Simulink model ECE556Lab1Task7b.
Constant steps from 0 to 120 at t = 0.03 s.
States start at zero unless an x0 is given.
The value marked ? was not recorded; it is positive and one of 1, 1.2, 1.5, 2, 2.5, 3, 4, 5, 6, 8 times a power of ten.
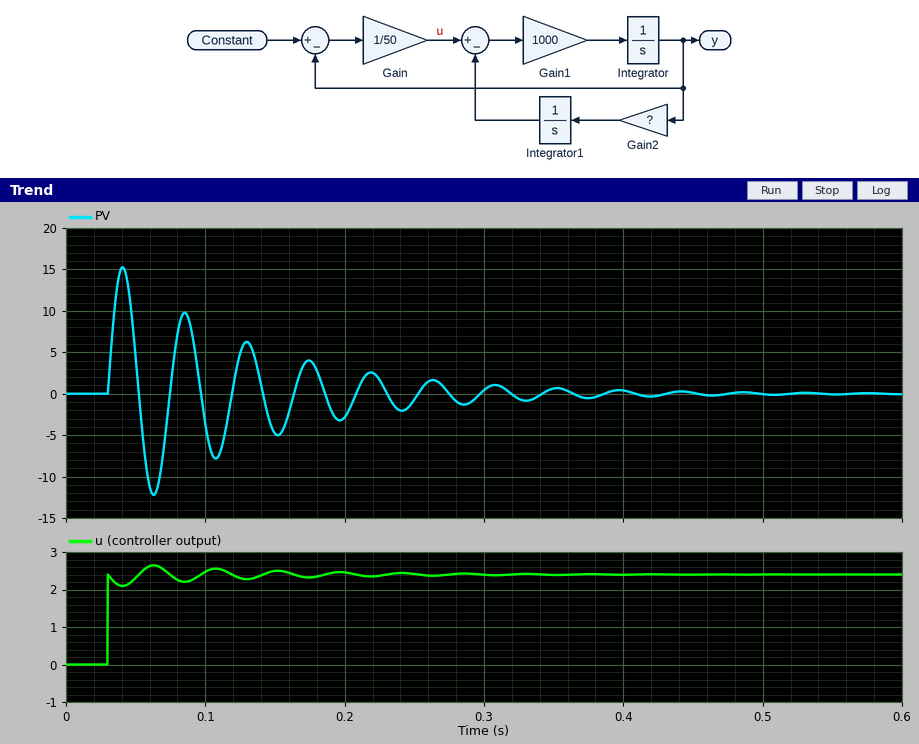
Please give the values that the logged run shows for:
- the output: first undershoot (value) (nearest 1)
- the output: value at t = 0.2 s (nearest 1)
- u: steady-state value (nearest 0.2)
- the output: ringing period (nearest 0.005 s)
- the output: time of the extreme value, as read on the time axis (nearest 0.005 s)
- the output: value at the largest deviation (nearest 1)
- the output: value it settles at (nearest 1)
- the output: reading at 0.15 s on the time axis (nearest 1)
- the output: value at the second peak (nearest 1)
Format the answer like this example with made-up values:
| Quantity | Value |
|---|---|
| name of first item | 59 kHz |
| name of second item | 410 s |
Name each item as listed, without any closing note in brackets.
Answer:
| Quantity | Value |
|---|---|
| the output: first undershoot (value) | -12 |
| the output: value at t = 0.2 s | -3 |
| u: steady-state value | 2.4 |
| the output: ringing period | 0.045 s |
| the output: time of the extreme value, as read on the time axis | 0.040 s |
| the output: value at the largest deviation | 15 |
| the output: value it settles at | 0 |
| the output: reading at 0.15 s on the time axis | -5 |
| the output: value at the second peak | 10 |
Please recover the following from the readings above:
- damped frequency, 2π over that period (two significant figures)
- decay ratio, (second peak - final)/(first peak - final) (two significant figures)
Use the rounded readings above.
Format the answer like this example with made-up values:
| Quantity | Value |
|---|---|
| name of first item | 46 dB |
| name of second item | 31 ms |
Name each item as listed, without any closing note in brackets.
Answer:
| Quantity | Value |
|---|---|
| damped frequency, 2π over that period | 140 rad/s |
| decay ratio, (second peak - final)/(first peak - final) | 0.67 |
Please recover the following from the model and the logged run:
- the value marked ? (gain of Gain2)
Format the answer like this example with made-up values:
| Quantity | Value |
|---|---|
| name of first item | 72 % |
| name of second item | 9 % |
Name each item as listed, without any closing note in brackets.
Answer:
| Quantity | Value |
|---|---|
| the value marked ? | 20 |
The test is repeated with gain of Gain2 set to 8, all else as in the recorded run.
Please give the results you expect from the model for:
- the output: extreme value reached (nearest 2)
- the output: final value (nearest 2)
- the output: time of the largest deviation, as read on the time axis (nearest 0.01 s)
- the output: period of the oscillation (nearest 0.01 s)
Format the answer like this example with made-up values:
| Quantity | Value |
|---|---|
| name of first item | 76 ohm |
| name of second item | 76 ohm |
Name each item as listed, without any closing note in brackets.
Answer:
| Quantity | Value |
|---|---|
| the output: extreme value reached | 22 |
| the output: final value | 0 |
| the output: time of the largest deviation, as read on the time axis | 0.05 s |
| the output: period of the oscillation | 0.07 s |
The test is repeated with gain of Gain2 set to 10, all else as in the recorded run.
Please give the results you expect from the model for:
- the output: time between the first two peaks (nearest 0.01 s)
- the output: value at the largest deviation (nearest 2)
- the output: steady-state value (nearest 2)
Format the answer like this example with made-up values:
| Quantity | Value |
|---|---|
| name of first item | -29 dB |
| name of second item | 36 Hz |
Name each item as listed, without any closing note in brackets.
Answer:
| Quantity | Value |
|---|---|
| the output: time between the first two peaks | 0.06 s |
| the output: value at the largest deviation | 20 |
| the output: steady-state value | 0 |
